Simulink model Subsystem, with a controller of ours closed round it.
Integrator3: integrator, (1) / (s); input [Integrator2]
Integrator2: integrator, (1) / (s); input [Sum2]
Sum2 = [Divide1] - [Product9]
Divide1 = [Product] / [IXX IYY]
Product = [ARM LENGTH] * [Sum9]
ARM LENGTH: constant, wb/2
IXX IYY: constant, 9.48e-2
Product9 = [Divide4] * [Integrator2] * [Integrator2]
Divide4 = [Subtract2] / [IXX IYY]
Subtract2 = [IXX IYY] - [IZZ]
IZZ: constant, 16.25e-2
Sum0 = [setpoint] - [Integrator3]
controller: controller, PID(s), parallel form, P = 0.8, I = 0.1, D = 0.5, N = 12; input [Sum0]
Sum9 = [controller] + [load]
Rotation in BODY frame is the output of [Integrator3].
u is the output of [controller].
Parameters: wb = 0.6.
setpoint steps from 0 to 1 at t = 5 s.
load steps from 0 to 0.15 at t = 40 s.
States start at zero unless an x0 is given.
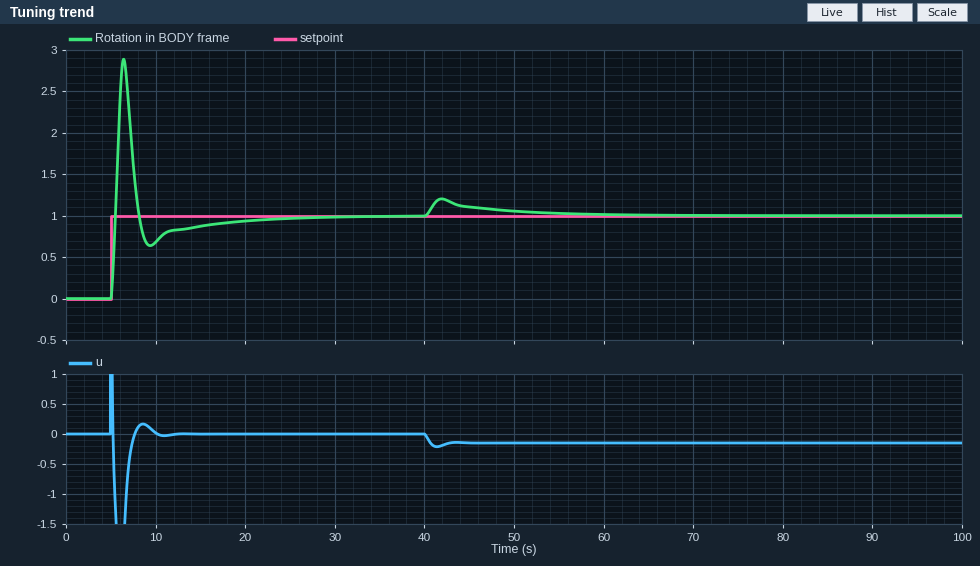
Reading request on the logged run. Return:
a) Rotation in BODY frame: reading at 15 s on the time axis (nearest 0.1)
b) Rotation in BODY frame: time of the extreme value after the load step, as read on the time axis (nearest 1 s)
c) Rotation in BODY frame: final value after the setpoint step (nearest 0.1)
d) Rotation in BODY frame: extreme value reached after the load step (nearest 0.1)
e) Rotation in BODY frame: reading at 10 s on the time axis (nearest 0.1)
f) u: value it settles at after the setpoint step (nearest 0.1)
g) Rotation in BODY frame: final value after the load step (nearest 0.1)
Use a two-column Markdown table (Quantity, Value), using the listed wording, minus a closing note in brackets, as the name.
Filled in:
| Quantity | Value |
|---|---|
| Rotation in BODY frame: reading at 15 s on the time axis | 0.9 |
| Rotation in BODY frame: time of the extreme value after the load step, as read on the time axis | 42 s |
| Rotation in BODY frame: final value after the setpoint step | 1.0 |
| Rotation in BODY frame: extreme value reached after the load step | 1.2 |
| Rotation in BODY frame: reading at 10 s on the time axis | 0.7 |
| u: value it settles at after the setpoint step | 0.0 |
| Rotation in BODY frame: final value after the load step | 1.0 |
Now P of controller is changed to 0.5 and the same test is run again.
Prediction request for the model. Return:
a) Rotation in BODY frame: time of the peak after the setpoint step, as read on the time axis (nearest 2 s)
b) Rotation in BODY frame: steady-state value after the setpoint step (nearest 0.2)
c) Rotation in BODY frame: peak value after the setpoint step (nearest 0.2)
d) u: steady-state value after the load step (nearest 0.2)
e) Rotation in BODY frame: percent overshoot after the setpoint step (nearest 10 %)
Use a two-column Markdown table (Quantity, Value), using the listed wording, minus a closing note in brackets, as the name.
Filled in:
| Quantity | Value |
|---|---|
| Rotation in BODY frame: time of the peak after the setpoint step, as read on the time axis | 6 s |
| Rotation in BODY frame: steady-state value after the setpoint step | 1.0 |
| Rotation in BODY frame: peak value after the setpoint step | 2.4 |
| u: steady-state value after the load step | -0.2 |
| Rotation in BODY frame: percent overshoot after the setpoint step | 150 % |
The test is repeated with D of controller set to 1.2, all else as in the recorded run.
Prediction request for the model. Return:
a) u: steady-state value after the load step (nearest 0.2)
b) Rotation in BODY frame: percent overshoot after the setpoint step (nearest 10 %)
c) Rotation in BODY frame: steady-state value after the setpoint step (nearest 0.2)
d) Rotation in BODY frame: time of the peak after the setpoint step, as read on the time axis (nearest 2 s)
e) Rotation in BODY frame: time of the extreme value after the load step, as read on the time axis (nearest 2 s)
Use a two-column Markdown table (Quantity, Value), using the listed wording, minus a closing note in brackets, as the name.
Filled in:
| Quantity | Value |
|---|---|
| u: steady-state value after the load step | -0.2 |
| Rotation in BODY frame: percent overshoot after the setpoint step | 130 % |
| Rotation in BODY frame: steady-state value after the setpoint step | 1.0 |
| Rotation in BODY frame: time of the peak after the setpoint step, as read on the time axis | 6 s |
| Rotation in BODY frame: time of the extreme value after the load step, as read on the time axis | 44 s |
